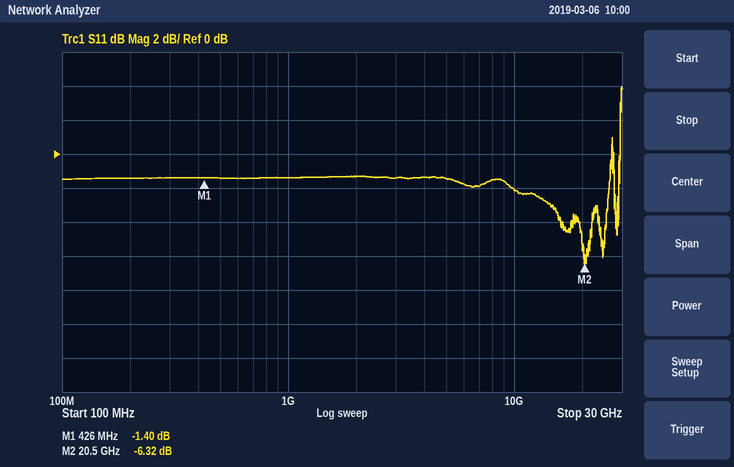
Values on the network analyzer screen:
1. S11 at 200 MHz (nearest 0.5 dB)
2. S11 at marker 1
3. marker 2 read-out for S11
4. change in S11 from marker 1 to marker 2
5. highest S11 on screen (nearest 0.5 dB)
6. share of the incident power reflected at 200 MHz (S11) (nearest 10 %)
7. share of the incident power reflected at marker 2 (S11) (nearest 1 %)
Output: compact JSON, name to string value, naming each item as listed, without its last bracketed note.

{"S11 at 200 MHz": "-1.5 dB", "S11 at marker 1": "-1.40 dB", "marker 2 read-out for S11": "-6.32 dB", "change in S11 from marker 1 to marker 2": "-4.92 dB", "highest S11 on screen": "4.0 dB", "share of the incident power reflected at 200 MHz (S11)": "70 %", "share of the incident power reflected at marker 2 (S11)": "23 %"}
